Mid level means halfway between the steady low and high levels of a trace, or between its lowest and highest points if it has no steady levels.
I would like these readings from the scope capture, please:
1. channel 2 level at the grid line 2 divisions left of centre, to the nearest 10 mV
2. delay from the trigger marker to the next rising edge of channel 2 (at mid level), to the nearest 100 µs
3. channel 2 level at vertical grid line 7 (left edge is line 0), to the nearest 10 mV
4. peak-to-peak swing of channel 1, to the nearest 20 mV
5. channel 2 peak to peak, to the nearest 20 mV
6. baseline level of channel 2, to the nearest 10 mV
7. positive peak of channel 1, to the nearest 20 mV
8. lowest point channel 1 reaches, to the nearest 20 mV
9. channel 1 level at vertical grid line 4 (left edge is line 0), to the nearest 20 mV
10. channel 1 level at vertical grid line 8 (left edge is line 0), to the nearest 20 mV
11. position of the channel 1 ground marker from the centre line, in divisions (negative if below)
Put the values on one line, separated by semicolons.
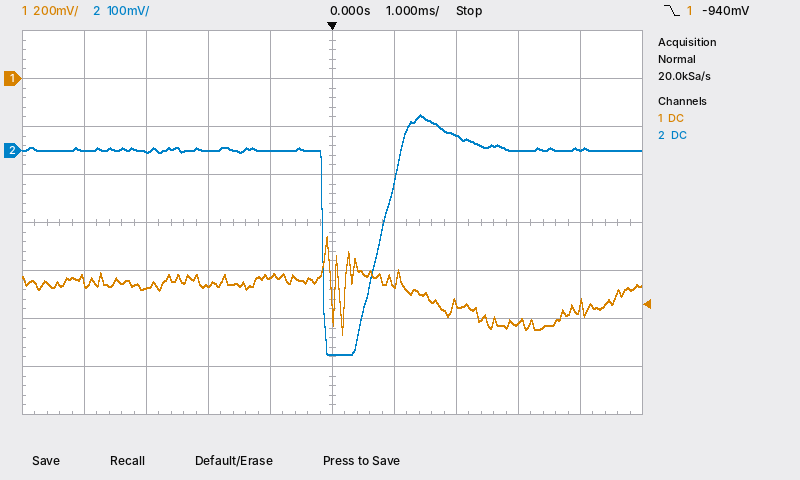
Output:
0 mV; 800 µs; 30 mV; 400 mV; 500 mV; 0 mV; -660 mV; -1.06 V; -820 mV; -1.02 V; +3.0 div
